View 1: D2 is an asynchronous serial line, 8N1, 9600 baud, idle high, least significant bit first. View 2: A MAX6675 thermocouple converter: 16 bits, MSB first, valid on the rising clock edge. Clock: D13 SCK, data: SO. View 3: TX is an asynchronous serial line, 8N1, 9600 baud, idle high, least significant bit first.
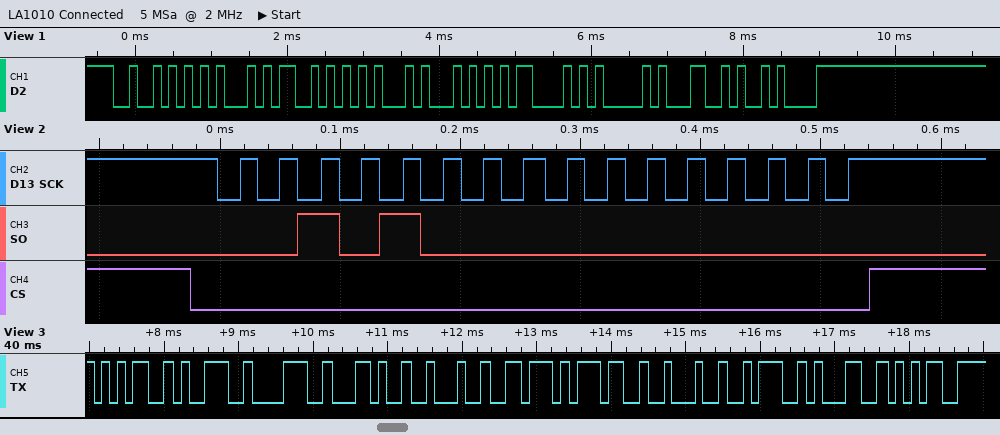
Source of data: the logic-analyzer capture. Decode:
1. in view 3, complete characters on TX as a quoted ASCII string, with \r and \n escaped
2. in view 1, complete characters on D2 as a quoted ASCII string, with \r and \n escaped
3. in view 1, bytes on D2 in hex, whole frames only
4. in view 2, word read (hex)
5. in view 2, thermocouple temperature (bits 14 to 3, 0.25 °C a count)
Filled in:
"598,\"v7\":15"
"RESETCAL\n"
52 45 53 45 54 43 41 4C 0A
0x2800
320.00 °C
